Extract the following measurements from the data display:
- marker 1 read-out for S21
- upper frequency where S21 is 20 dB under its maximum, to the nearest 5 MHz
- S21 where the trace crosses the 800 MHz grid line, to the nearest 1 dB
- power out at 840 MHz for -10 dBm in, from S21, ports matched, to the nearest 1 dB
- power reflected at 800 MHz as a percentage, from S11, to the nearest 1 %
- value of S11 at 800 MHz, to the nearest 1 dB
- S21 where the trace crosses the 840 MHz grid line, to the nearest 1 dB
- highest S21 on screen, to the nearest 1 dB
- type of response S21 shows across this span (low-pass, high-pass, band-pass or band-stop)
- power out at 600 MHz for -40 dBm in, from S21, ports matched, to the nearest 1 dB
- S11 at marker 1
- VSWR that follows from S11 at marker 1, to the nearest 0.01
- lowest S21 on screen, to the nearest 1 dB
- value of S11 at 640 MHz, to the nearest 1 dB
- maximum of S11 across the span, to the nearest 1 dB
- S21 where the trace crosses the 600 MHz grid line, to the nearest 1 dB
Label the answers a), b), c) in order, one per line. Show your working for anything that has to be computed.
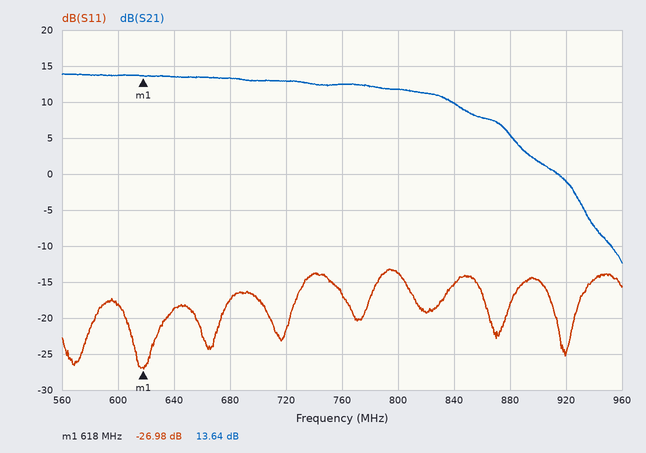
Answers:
a) 13.64 dB
b) 935 MHz
c) 12 dB
d) -10 dBm + (10 dB) = 0 dBm
e) 10^(-14/10) ≈ 4 %
f) -14 dB
g) 10 dB
h) 14 dB
i) low-pass
j) -40 dBm + (14 dB) = -26 dBm
k) -26.98 dB
l) (1 + 0.0448)/(1 − 0.0448) ≈ 1.09
m) -12 dB
n) -19 dB
o) -13 dB
p) 14 dB
